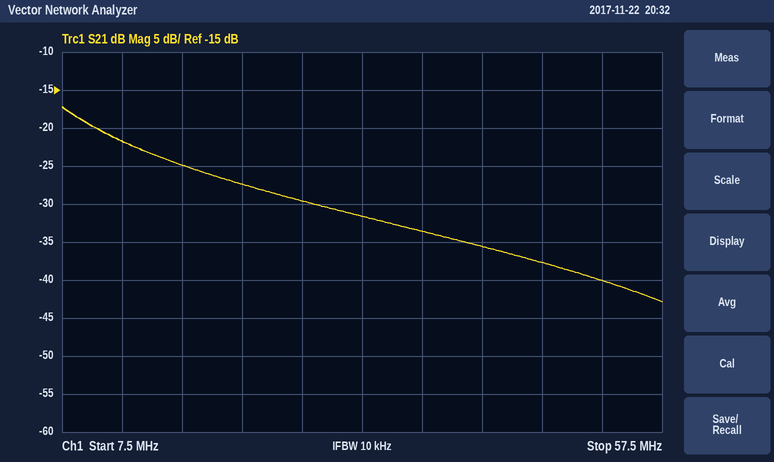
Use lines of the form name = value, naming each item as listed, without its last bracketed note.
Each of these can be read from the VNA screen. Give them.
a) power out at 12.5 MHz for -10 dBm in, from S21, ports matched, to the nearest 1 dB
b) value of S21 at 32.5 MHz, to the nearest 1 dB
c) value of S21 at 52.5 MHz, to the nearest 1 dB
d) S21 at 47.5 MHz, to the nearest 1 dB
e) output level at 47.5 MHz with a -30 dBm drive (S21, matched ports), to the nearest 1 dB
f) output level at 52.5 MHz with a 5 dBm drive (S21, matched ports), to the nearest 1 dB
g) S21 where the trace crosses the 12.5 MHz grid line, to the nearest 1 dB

power out at 12.5 MHz for -10 dBm in, from S21, ports matched, to the nearest 1 dB = -32 dBm
value of S21 at 32.5 MHz, to the nearest 1 dB = -32 dB
value of S21 at 52.5 MHz, to the nearest 1 dB = -40 dB
S21 at 47.5 MHz, to the nearest 1 dB = -38 dB
output level at 47.5 MHz with a -30 dBm drive (S21, matched ports), to the nearest 1 dB = -68 dBm
output level at 52.5 MHz with a 5 dBm drive (S21, matched ports), to the nearest 1 dB = -35 dBm
S21 where the trace crosses the 12.5 MHz grid line, to the nearest 1 dB = -22 dB
